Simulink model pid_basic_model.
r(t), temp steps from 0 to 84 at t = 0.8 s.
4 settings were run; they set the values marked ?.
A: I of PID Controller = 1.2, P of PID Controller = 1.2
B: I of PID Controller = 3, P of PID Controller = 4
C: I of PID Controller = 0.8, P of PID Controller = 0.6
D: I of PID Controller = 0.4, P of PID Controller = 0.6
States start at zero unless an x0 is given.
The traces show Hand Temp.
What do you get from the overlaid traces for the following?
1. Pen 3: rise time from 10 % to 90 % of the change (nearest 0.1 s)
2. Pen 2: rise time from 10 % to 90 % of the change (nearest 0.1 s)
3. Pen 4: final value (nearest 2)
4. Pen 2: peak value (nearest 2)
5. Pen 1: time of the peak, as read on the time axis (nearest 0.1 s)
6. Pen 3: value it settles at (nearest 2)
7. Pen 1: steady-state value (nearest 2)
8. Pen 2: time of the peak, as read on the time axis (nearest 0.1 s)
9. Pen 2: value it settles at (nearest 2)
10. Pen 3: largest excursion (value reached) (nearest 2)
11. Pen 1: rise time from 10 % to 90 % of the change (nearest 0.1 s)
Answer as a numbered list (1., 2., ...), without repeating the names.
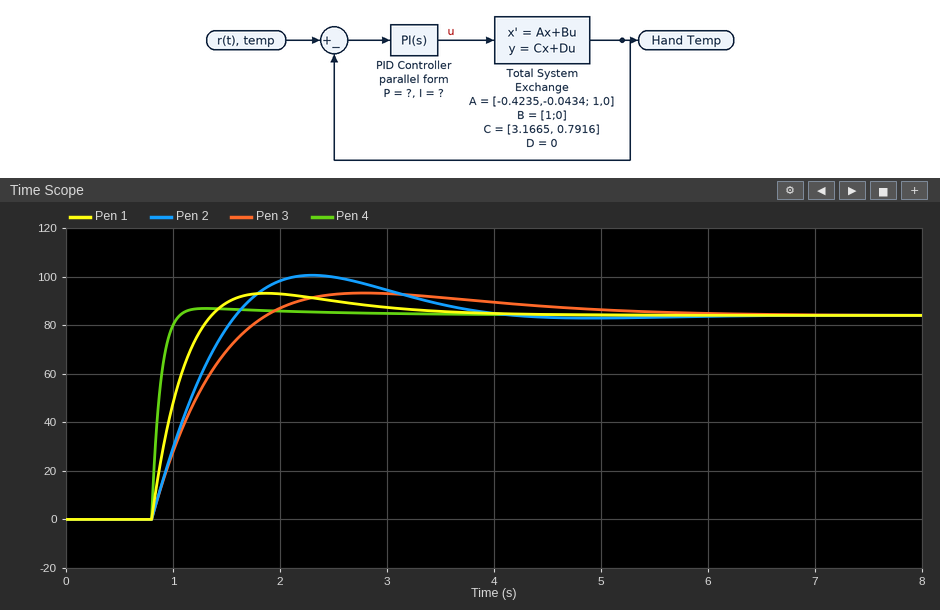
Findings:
1. 0.8 s
2. 0.6 s
3. 84
4. 100
5. 1.9 s
6. 84
7. 84
8. 2.3 s
9. 84
10. 94
11. 0.4 s
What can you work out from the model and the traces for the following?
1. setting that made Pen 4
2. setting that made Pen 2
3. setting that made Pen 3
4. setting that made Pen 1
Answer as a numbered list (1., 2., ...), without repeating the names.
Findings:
1. B
2. C
3. D
4. A
